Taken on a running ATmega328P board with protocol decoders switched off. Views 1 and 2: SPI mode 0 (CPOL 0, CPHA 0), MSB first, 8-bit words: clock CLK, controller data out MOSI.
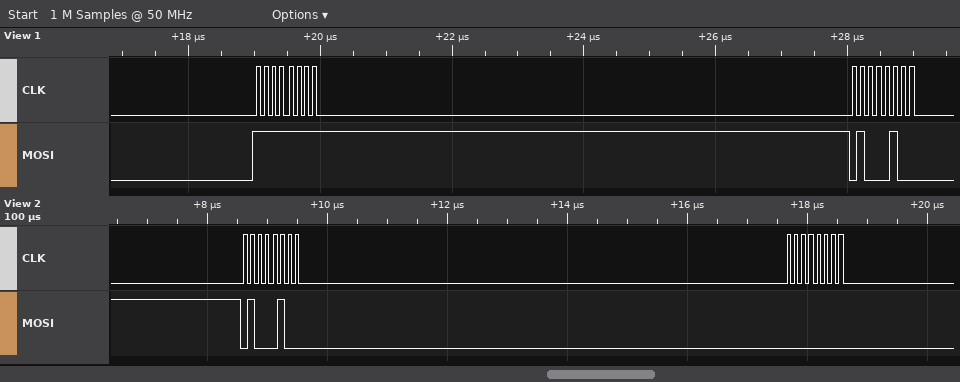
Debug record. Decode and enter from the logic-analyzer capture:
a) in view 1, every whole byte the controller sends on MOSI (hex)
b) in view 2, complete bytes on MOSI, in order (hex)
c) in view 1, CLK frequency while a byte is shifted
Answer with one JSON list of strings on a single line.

["0xFF 0x44", "44 00", "8 MHz"]
